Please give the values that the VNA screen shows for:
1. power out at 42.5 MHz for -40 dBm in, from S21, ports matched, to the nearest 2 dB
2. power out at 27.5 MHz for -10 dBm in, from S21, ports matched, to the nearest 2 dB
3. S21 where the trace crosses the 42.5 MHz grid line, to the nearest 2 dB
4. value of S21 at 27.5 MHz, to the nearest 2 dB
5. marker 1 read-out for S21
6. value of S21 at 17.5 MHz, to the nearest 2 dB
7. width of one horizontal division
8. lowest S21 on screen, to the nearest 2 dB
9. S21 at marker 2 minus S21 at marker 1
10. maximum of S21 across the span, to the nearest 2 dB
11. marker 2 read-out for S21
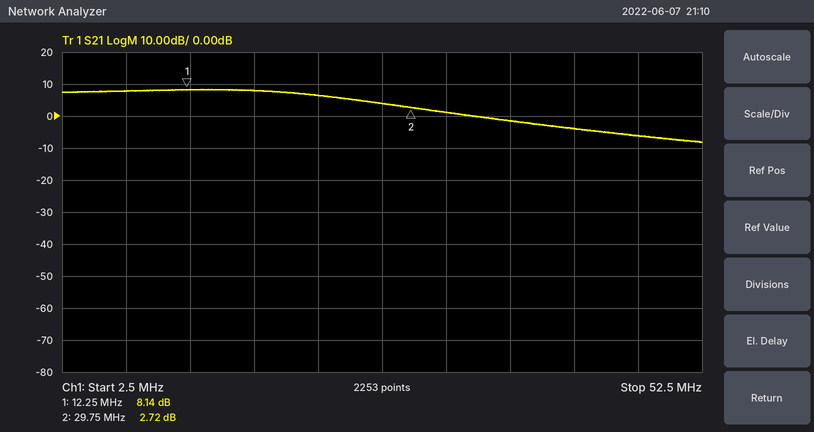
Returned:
-44 dBm
-6 dBm
-4 dB
4 dB
8.14 dB
8 dB
5 MHz
-8 dB
-5.42 dB
8 dB
2.72 dB
